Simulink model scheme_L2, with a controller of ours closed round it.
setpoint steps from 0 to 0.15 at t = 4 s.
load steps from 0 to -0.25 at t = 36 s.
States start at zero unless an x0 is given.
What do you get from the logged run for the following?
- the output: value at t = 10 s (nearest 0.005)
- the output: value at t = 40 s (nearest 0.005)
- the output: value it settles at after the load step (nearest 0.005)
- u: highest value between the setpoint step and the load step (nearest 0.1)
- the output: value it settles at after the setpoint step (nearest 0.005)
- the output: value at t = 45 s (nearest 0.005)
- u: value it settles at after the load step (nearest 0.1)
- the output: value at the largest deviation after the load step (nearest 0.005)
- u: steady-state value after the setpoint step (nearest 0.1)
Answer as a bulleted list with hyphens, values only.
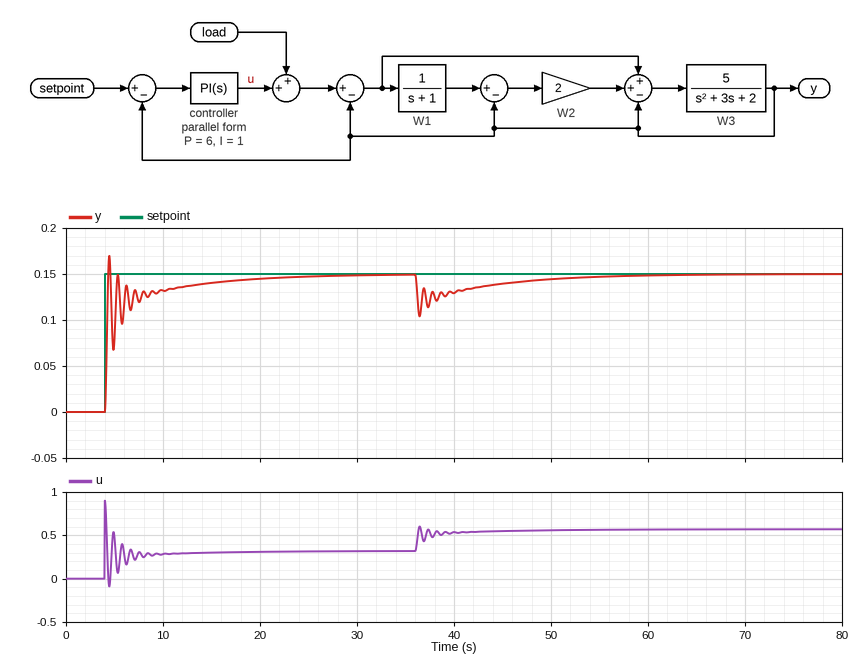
- 0.130
- 0.130
- 0.150
- 0.9
- 0.150
- 0.140
- 0.6
- 0.105
- 0.3
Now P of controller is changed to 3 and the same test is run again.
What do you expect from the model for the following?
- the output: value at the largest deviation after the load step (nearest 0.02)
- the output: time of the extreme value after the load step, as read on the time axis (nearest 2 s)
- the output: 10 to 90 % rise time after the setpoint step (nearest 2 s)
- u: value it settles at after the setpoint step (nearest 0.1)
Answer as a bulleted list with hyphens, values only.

- 0.08
- 36 s
- 6 s
- 0.3
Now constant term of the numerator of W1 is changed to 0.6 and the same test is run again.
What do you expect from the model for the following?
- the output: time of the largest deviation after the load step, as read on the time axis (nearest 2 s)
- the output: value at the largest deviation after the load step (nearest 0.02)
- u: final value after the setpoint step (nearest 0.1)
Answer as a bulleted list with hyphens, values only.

- 36 s
- 0.10
- 0.4
